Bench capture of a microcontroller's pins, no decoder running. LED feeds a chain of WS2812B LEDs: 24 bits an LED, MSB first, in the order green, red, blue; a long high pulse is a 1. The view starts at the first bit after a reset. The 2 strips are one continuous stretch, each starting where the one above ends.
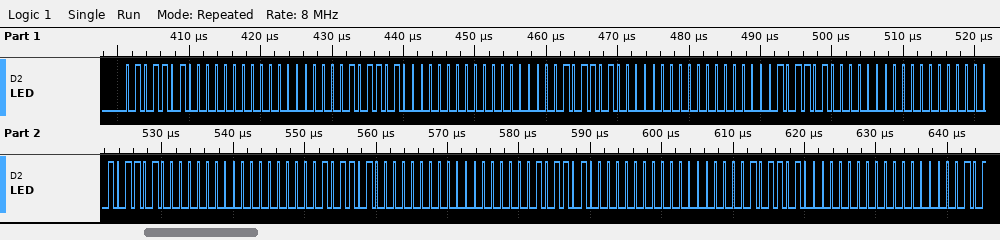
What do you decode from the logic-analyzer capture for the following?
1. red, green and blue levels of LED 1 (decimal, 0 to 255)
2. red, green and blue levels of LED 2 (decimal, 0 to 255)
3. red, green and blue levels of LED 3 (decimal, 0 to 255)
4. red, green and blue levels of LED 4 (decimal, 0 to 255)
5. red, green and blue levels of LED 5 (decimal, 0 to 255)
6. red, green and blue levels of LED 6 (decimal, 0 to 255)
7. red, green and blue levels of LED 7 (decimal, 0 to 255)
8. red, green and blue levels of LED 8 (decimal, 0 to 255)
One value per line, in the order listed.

0, 90, 0
0, 90, 0
0, 90, 0
0, 90, 0
0, 90, 0
0, 90, 0
0, 90, 0
0, 90, 0
